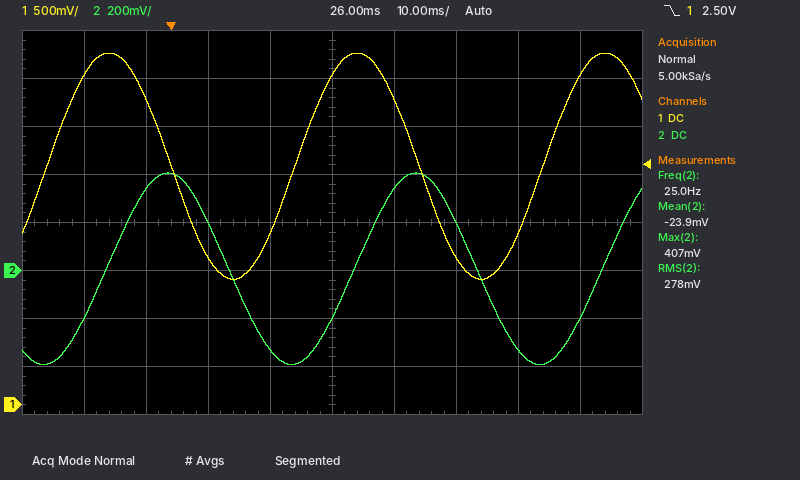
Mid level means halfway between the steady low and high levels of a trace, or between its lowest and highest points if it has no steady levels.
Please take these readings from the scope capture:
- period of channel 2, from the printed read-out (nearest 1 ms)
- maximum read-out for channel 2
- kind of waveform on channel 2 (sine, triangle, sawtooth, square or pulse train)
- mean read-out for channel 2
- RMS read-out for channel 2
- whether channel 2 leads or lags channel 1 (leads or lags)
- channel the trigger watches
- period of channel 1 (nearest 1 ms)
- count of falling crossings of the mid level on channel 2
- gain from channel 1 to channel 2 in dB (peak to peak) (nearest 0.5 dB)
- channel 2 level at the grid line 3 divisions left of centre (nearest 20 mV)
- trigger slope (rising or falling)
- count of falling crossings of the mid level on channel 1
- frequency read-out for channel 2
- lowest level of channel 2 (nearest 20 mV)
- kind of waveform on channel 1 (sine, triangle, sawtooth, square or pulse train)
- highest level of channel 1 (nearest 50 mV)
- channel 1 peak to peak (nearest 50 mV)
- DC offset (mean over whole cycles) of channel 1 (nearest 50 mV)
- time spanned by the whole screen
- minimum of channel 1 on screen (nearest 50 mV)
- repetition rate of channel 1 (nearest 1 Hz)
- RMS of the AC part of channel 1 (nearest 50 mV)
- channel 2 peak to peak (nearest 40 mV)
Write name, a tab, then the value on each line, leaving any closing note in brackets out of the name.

period of channel 2, from the printed read-out	40 ms
maximum read-out for channel 2	407 mV
kind of waveform on channel 2	sine
mean read-out for channel 2	-23.9 mV
RMS read-out for channel 2	278 mV
whether channel 2 leads or lags channel 1	lags
channel the trigger watches	channel 1
period of channel 1	40 ms
count of falling crossings of the mid level on channel 2	2
gain from channel 1 to channel 2 in dB (peak to peak)	-9.5 dB
channel 2 level at the grid line 3 divisions left of centre	340 mV
trigger slope	falling
count of falling crossings of the mid level on channel 1	2
frequency read-out for channel 2	25.0 Hz
lowest level of channel 2	-400 mV
kind of waveform on channel 1	sine
highest level of channel 1	3.65 V
channel 1 peak to peak	2.35 V
DC offset (mean over whole cycles) of channel 1	2.50 V
time spanned by the whole screen	100 ms
minimum of channel 1 on screen	1.30 V
repetition rate of channel 1	25 Hz
RMS of the AC part of channel 1	850 mV
channel 2 peak to peak	800 mV
